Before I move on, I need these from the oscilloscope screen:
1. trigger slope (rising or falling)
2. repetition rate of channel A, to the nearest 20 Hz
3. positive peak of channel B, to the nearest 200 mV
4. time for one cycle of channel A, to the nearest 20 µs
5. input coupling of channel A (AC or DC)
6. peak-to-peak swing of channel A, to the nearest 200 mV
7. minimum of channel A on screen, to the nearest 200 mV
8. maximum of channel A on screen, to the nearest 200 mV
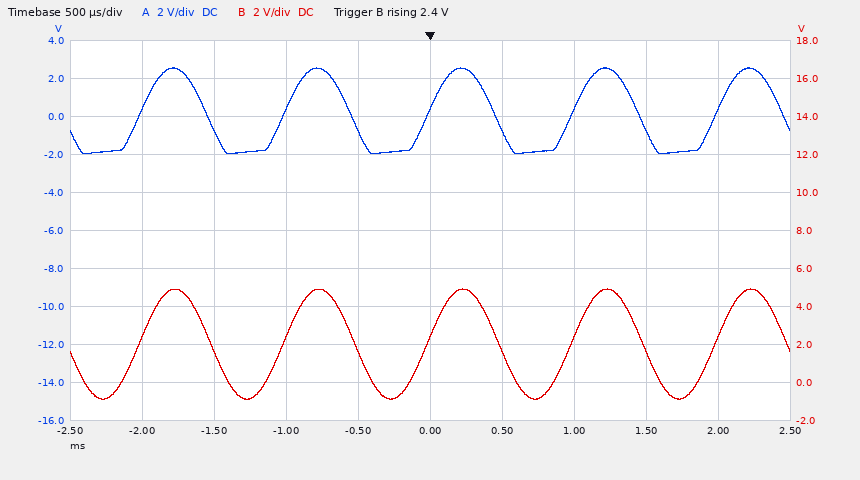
rising
1.00 kHz
5.0 V
1.00 ms
DC
4.6 V
-2.0 V
2.6 V
